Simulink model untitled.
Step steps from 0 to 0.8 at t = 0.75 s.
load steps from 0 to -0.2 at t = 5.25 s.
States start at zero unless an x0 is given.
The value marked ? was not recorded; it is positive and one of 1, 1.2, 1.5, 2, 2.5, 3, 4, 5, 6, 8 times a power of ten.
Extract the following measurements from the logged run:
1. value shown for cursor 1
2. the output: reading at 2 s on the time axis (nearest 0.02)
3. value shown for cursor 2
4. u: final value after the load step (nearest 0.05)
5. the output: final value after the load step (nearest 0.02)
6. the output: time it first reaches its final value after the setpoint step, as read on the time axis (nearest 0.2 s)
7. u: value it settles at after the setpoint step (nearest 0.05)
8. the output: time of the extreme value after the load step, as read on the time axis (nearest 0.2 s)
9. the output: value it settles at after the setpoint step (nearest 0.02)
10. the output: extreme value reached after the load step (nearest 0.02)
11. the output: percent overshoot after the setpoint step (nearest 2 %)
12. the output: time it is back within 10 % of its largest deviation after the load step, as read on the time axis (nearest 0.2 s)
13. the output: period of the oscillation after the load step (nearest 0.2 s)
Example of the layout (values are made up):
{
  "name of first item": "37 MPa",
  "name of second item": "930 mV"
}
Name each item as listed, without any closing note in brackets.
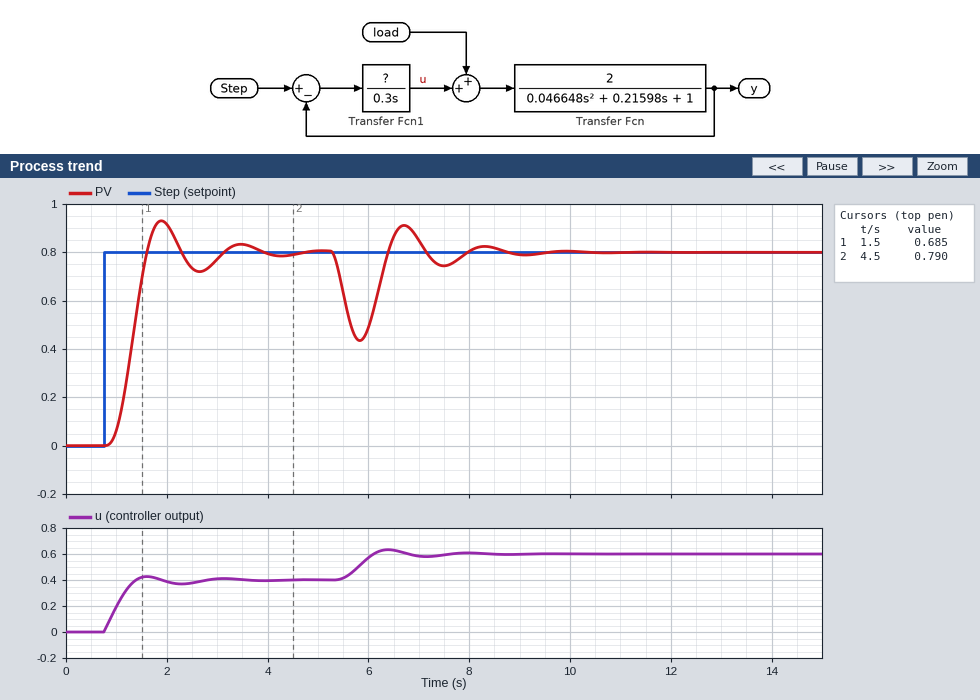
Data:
{
  "value shown for cursor 1": "0.685",
  "the output: reading at 2 s on the time axis": "0.92",
  "value shown for cursor 2": "0.790",
  "u: final value after the load step": "0.60",
  "the output: final value after the load step": "0.80",
  "the output: time it first reaches its final value after the setpoint step, as read on the time axis": "1.6 s",
  "u: value it settles at after the setpoint step": "0.40",
  "the output: time of the extreme value after the load step, as read on the time axis": "5.8 s",
  "the output: value it settles at after the setpoint step": "0.80",
  "the output: extreme value reached after the load step": "0.44",
  "the output: percent overshoot after the setpoint step": "16 %",
  "the output: time it is back within 10 % of its largest deviation after the load step, as read on the time axis": "7.8 s",
  "the output: period of the oscillation after the load step": "1.6 s"
}
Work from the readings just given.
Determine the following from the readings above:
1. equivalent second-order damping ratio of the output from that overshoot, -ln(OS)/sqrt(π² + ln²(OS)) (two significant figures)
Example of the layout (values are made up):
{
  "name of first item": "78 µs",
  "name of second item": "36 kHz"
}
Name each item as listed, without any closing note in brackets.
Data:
{
  "equivalent second-order damping ratio of the output from that overshoot, -ln(OS)/sqrt(π² + ln²(OS))": "0.50"
}
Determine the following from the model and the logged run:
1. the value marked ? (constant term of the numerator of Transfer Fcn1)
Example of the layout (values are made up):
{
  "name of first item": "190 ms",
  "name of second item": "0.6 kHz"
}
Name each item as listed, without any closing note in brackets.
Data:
{
  "the value marked ?": "0.3"
}
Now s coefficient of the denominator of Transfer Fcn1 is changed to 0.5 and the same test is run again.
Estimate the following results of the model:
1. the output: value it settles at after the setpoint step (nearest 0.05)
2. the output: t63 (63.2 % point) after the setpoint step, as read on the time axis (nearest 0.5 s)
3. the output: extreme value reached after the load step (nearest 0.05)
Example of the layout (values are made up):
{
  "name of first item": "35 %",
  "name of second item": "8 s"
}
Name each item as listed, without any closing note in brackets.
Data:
{
  "the output: value it settles at after the setpoint step": "0.80",
  "the output: t63 (63.2 % point) after the setpoint step, as read on the time axis": "1.5 s",
  "the output: extreme value reached after the load step": "0.40"
}
